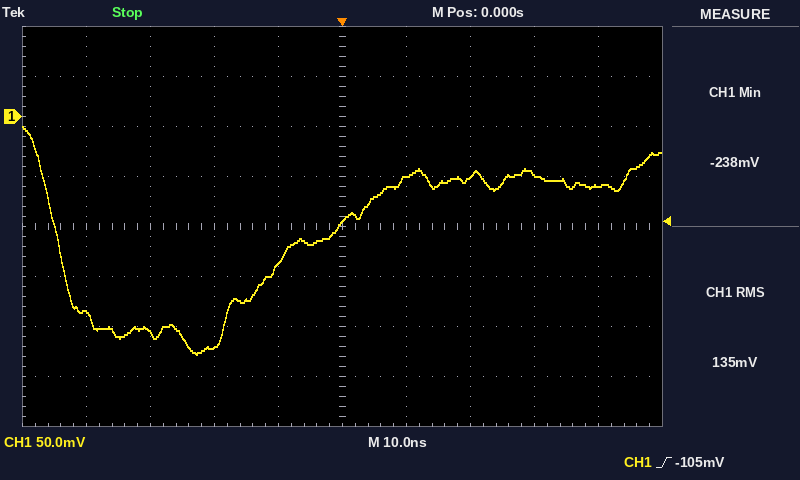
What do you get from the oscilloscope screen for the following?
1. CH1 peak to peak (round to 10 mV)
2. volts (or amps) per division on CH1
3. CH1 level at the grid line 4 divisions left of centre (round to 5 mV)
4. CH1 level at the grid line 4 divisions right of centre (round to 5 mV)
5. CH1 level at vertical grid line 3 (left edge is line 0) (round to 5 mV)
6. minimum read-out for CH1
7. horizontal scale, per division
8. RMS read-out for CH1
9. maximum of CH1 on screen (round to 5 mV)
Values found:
230 mV
50 mV
-195 mV
-70 mV
-230 mV
-238 mV
10 ns
135 mV
-10 mV
